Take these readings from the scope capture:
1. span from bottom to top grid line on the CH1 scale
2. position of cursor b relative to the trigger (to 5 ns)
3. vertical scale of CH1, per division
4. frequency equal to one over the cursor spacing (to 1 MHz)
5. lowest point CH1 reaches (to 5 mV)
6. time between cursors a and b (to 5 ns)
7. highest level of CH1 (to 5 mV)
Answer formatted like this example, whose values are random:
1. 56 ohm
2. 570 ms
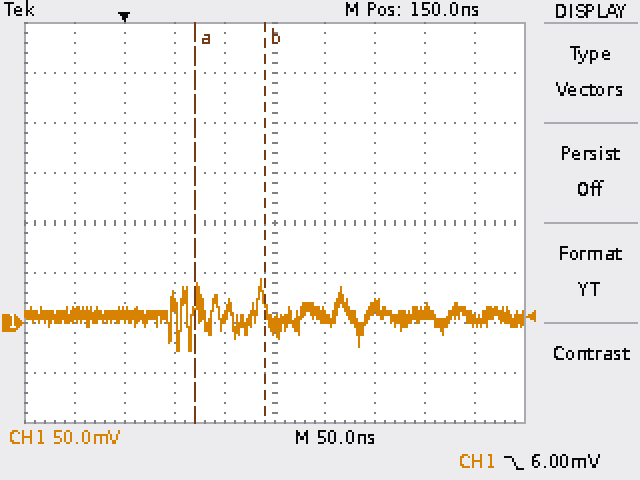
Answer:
1. 400 mV
2. +140 ns
3. 50 mV
4. 14 MHz
5. -30 mV
6. 70 ns
7. 45 mV
